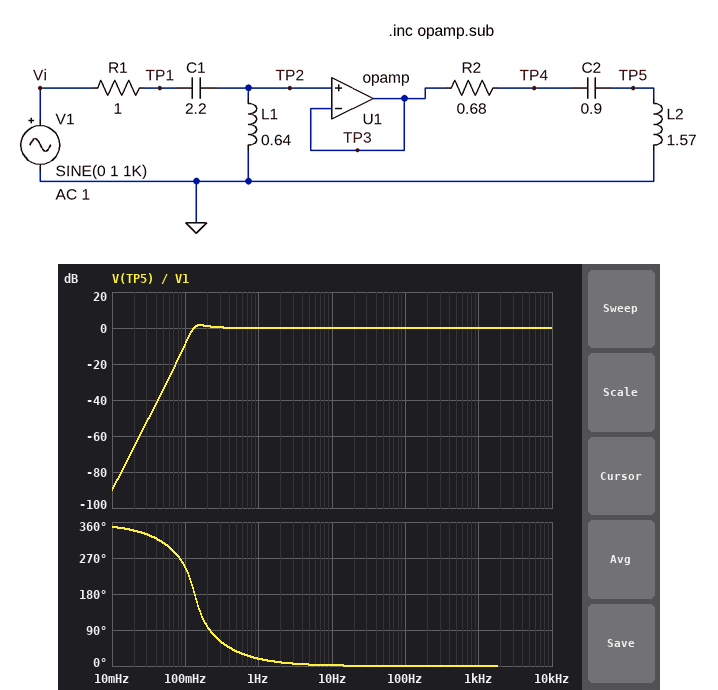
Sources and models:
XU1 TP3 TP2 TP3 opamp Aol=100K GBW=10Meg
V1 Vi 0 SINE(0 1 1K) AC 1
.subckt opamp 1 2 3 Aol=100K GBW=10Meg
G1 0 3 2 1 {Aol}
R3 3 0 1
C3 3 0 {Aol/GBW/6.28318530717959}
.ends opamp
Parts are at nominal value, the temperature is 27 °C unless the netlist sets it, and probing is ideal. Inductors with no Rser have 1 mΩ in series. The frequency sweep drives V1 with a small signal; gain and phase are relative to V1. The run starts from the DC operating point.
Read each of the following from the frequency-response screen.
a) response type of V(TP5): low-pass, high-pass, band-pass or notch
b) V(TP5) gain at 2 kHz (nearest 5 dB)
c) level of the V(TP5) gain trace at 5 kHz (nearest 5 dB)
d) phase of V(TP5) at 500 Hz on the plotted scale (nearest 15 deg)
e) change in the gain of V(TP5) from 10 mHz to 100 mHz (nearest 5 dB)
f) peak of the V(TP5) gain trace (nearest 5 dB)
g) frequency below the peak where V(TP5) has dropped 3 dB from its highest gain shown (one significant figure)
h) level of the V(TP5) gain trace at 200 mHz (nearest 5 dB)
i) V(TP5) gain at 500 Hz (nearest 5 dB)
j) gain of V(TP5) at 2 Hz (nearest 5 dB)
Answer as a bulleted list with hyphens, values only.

- high-pass
- 0 dB
- 0 dB
- 0 deg
- 80 dB
- 0 dB
- 100 mHz
- 0 dB
- 0 dB
- 0 dB
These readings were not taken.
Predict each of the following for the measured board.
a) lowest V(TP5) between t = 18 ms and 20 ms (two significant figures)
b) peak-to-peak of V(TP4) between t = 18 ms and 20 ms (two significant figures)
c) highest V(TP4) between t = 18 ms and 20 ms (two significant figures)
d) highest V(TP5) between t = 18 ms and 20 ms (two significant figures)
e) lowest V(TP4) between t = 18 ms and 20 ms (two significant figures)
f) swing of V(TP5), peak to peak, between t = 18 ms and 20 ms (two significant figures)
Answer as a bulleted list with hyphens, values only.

- -1.0 V
- 2.0 V
- 1.0 V
- 1.0 V
- -1.0 V
- 2.0 V
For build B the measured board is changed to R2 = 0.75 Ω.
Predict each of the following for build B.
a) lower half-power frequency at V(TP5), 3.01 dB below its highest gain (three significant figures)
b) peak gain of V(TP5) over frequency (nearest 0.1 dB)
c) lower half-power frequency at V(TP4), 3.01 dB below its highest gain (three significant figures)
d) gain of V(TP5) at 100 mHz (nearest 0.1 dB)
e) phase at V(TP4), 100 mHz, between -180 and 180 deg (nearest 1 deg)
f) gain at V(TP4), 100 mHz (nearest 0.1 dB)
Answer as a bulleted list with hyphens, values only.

- 125 mHz
- 1.0 dB
- 231 mHz
- -9.2 dB
- 64 deg
- -11.2 dB
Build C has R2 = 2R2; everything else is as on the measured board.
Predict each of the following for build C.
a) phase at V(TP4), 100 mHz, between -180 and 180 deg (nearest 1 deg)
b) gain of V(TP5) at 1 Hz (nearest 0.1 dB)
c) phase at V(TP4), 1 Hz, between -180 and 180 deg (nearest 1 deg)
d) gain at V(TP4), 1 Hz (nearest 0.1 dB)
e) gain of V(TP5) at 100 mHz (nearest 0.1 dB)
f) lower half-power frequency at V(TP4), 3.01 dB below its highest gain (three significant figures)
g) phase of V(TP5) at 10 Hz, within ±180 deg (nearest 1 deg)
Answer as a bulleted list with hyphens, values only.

- 37 deg
- -0.2 dB
- 27 deg
- -0.3 dB
- -15.8 dB
- 340 mHz
- 3 deg
